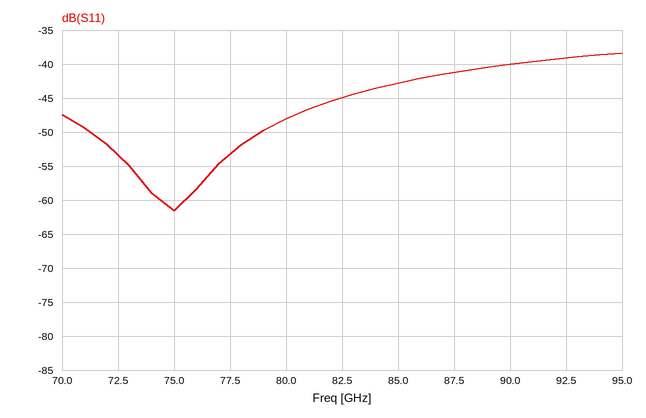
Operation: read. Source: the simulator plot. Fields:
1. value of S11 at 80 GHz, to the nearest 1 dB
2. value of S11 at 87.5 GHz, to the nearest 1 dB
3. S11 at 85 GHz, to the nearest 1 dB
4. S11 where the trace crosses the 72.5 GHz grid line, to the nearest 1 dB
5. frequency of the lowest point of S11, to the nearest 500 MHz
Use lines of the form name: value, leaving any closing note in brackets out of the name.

value of S11 at 80 GHz, to the nearest 1 dB: -48 dB
value of S11 at 87.5 GHz, to the nearest 1 dB: -41 dB
S11 at 85 GHz, to the nearest 1 dB: -43 dB
S11 where the trace crosses the 72.5 GHz grid line, to the nearest 1 dB: -53 dB
frequency of the lowest point of S11, to the nearest 500 MHz: 75.0 GHz
